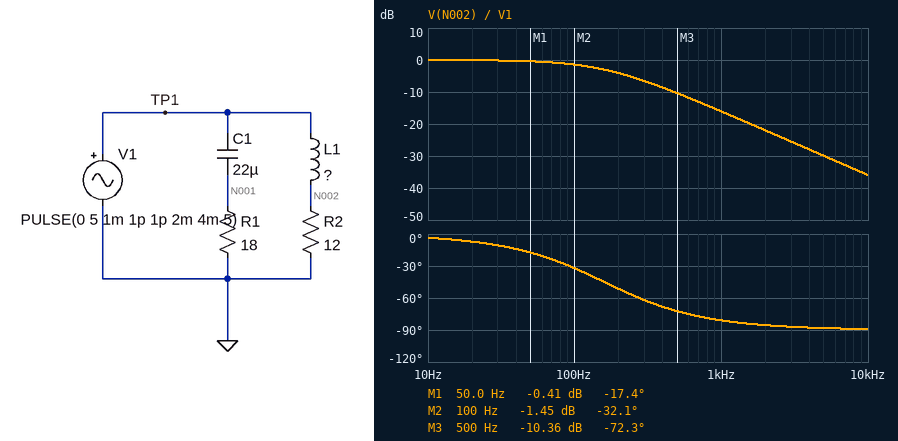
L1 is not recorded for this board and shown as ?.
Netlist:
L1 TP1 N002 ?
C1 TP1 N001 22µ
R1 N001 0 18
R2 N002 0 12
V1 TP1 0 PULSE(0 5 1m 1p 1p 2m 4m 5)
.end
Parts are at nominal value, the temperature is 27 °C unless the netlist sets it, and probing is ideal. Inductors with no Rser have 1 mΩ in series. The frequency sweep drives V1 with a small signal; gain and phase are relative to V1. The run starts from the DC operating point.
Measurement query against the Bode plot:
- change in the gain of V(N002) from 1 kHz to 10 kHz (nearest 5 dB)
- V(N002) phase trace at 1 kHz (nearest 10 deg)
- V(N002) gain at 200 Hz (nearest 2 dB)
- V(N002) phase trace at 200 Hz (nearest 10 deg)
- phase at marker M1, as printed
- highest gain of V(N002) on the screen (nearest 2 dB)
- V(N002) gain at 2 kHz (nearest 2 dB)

-20 dB
-80 deg
-4 dB
-50 deg
-17.4 deg
0 dB
-22 dB
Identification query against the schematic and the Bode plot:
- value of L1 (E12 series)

12 mH
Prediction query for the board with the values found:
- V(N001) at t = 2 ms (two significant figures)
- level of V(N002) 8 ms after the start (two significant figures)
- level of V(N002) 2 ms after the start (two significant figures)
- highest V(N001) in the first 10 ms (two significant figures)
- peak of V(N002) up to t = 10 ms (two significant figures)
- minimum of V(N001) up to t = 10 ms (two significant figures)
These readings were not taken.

400 mV
1.6 V
3.2 V
5.0 V
4.4 V
-5.0 V
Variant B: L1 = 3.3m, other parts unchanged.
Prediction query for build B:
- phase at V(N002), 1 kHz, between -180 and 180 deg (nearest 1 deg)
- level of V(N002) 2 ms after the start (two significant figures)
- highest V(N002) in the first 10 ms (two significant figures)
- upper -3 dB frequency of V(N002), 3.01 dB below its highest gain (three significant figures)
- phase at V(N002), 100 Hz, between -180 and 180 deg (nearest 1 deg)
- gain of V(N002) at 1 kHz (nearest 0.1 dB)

-60 deg
4.9 V
5.0 V
579 Hz
-10 deg
-6.0 dB
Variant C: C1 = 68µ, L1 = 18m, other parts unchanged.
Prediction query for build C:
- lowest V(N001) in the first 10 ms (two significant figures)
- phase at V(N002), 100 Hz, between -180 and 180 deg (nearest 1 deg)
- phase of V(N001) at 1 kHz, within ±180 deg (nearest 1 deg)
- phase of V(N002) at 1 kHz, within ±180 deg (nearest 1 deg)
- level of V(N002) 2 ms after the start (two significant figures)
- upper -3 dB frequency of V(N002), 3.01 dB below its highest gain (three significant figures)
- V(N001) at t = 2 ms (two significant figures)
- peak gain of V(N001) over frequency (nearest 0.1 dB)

-4.2 V
-43 deg
7 deg
-84 deg
2.4 V
106 Hz
2.2 V
0 dB
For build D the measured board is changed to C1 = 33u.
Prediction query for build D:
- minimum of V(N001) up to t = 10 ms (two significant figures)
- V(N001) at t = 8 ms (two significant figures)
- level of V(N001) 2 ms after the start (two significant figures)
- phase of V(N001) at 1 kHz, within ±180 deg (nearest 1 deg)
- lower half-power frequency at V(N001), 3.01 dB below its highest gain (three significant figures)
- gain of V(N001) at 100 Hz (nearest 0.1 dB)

-4.8 V
-900 mV
930 mV
15 deg
268 Hz
-9.1 dB
